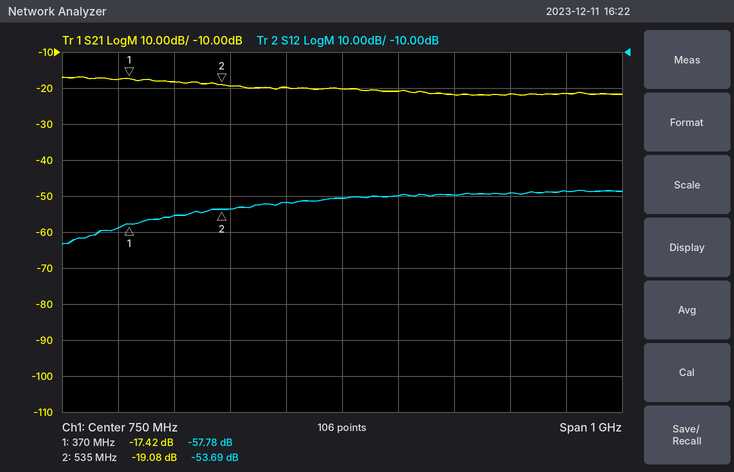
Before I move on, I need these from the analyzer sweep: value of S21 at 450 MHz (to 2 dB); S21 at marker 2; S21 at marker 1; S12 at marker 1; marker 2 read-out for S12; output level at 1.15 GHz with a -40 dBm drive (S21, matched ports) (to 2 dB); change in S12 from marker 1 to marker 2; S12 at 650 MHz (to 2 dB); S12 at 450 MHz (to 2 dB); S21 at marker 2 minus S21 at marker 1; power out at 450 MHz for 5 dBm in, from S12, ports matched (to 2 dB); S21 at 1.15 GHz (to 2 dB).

-18 dB
-19.08 dB
-17.42 dB
-57.78 dB
-53.69 dB
-62 dBm
4.09 dB
-52 dB
-56 dB
-1.66 dB
-50 dBm
-22 dB
